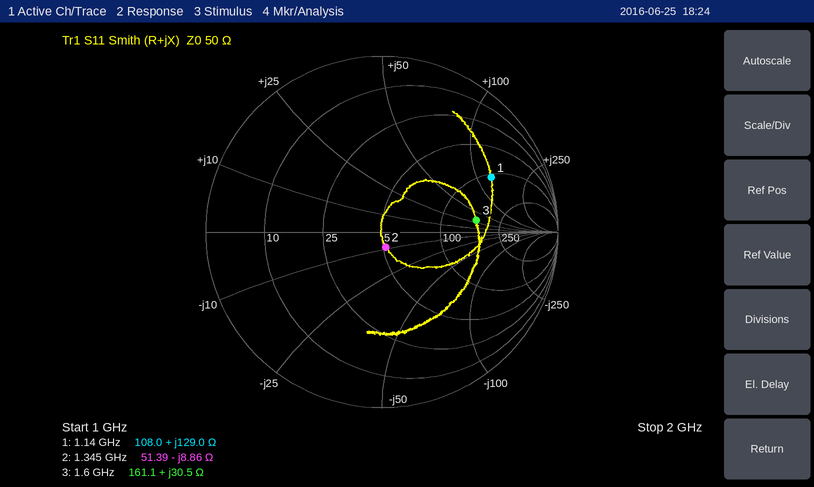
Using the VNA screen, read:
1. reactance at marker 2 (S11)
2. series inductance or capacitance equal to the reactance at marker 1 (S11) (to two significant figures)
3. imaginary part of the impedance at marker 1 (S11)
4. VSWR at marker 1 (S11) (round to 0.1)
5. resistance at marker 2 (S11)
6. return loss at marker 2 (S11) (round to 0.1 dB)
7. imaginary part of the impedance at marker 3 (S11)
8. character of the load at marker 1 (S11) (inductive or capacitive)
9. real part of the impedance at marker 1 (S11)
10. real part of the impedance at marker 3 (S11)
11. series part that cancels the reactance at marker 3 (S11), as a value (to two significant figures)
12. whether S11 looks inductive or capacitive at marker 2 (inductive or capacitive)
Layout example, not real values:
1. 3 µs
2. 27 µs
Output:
1. -8.86 Ω
2. 18 nH
3. +129.0 Ω
4. 5.5
5. 51.39 Ω
6. 21.1 dB
7. +30.5 Ω
8. inductive
9. 108.0 Ω
10. 161.1 Ω
11. 3.3 pF
12. capacitive
